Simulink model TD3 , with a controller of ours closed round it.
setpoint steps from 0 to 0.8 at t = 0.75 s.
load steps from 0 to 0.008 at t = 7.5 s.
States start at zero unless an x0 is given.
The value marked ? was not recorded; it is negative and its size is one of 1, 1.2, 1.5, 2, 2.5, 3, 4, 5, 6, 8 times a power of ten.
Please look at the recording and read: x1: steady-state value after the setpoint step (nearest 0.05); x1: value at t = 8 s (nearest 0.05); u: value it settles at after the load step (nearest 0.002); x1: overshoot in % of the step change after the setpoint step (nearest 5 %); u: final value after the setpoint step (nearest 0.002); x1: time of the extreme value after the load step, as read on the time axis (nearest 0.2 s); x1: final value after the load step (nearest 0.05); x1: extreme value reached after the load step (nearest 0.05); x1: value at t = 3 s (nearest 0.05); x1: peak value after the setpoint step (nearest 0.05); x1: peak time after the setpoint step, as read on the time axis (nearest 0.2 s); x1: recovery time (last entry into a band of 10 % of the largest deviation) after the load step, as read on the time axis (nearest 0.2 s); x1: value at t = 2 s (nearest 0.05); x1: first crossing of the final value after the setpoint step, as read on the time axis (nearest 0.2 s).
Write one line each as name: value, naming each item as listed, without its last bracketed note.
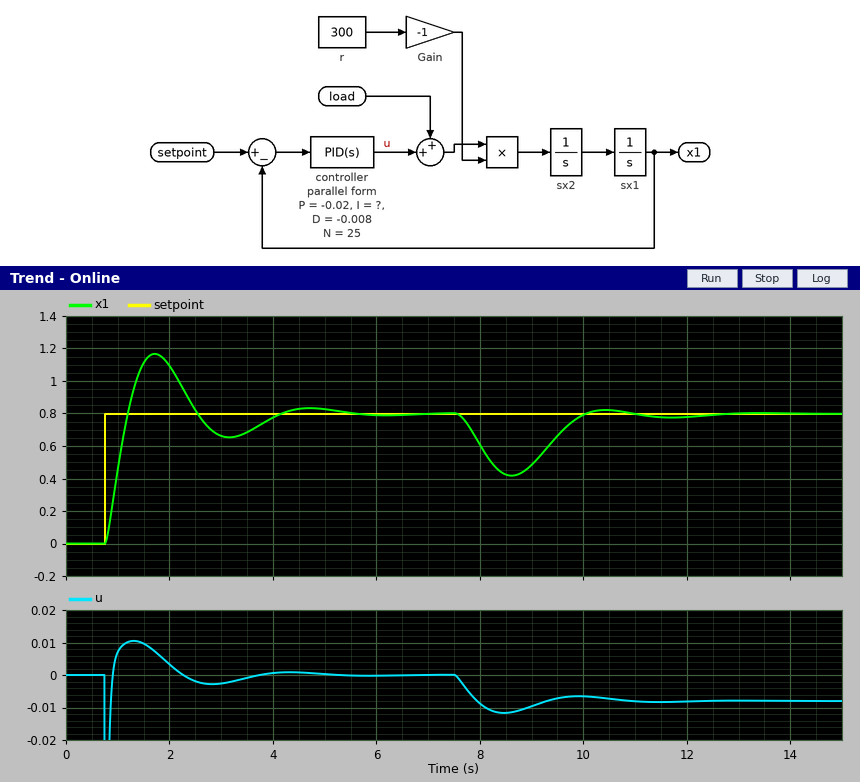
x1: steady-state value after the setpoint step: 0.80
x1: value at t = 8 s: 0.60
u: value it settles at after the load step: -0.008
x1: overshoot in % of the step change after the setpoint step: 45 %
u: final value after the setpoint step: 0.000
x1: time of the extreme value after the load step, as read on the time axis: 8.6 s
x1: final value after the load step: 0.80
x1: extreme value reached after the load step: 0.40
x1: value at t = 3 s: 0.65
x1: peak value after the setpoint step: 1.15
x1: peak time after the setpoint step, as read on the time axis: 1.8 s
x1: recovery time (last entry into a band of 10 % of the largest deviation) after the load step, as read on the time axis: 9.8 s
x1: value at t = 2 s: 1.10
x1: first crossing of the final value after the setpoint step, as read on the time axis: 1.2 s
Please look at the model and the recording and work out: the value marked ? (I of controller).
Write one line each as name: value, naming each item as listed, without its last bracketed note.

the value marked ?: -0.015
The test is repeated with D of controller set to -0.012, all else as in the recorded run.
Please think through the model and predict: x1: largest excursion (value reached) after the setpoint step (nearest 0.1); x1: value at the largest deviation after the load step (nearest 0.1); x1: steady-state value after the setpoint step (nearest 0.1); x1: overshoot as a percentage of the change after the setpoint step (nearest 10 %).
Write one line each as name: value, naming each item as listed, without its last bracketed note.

x1: largest excursion (value reached) after the setpoint step: 1.0
x1: value at the largest deviation after the load step: 0.5
x1: steady-state value after the setpoint step: 0.8
x1: overshoot as a percentage of the change after the setpoint step: 30 %
